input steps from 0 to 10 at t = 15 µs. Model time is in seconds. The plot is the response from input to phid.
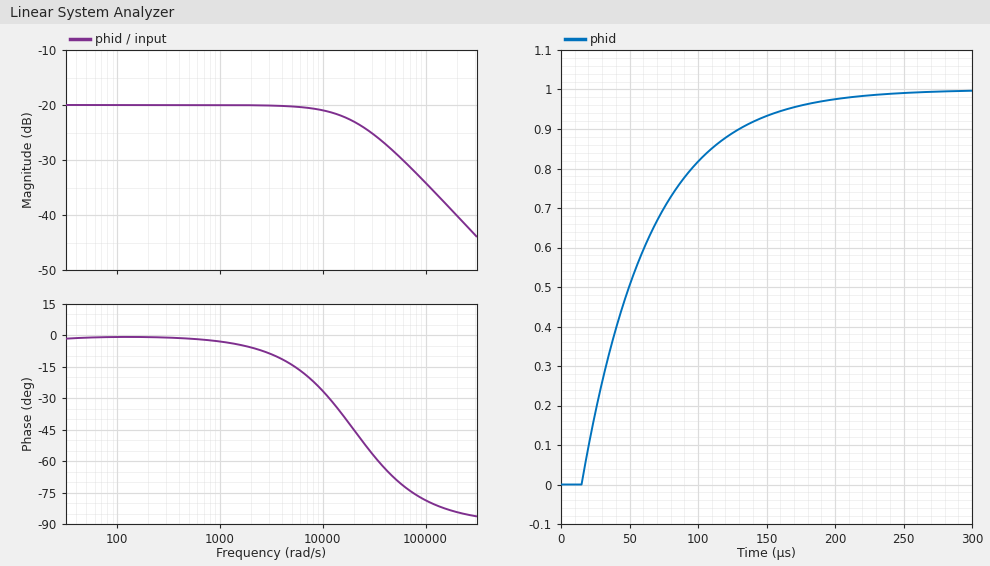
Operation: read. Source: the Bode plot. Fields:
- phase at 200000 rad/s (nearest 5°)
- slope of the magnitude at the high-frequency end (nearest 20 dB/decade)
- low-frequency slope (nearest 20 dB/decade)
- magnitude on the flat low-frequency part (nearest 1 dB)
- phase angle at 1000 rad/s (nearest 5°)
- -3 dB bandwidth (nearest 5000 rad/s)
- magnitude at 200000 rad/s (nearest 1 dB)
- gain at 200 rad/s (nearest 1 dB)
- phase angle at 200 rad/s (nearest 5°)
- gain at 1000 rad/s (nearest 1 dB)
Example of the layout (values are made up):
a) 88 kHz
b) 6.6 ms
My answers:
a) -85°
b) -20 dB/decade
c) 0 dB/decade
d) -20 dB
e) -5°
f) 20000 rad/s
g) -40 dB
h) -20 dB
i) 0°
j) -20 dB
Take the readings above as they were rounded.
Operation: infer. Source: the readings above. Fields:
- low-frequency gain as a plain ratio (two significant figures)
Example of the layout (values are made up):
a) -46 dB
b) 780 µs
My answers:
a) 0.10
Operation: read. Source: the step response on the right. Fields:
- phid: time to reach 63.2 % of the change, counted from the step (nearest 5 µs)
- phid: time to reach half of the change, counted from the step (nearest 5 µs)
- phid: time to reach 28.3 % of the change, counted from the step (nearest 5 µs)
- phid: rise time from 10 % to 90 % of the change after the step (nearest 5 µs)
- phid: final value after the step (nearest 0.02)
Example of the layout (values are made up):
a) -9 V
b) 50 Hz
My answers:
a) 50 µs
b) 35 µs
c) 15 µs
d) 110 µs
e) 1.00
